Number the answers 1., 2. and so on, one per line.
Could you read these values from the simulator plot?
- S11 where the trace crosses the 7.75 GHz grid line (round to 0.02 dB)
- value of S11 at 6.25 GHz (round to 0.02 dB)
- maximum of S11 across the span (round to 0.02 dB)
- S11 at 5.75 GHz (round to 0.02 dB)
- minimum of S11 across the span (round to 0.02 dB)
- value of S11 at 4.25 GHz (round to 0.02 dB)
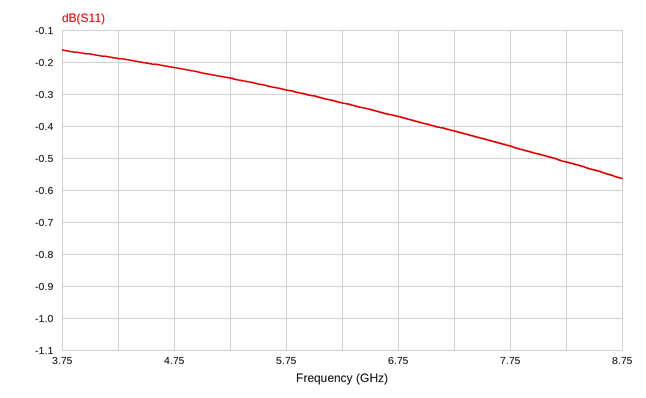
1. -0.46 dB
2. -0.32 dB
3. -0.16 dB
4. -0.28 dB
5. -0.56 dB
6. -0.18 dB
